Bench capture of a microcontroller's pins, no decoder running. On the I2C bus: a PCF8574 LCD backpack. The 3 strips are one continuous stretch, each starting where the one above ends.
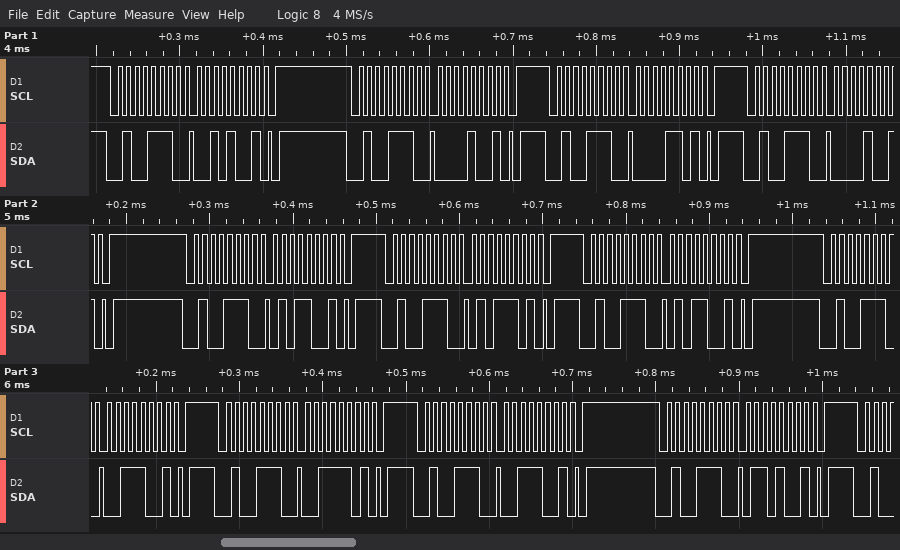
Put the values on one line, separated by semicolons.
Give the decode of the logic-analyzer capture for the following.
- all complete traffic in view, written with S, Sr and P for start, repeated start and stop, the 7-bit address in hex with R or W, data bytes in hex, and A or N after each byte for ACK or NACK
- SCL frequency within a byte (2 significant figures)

S 27W A 29 A P S 27W A 09 A P S 27W A 0D A P S 27W A 09 A P S 27W A 59 A P S 27W A 5D A P S 27W A 59 A P S 27W A 39 A P S 27W A 3D A P S 27W A 39 A P S 27W A 69 A P; 100 kHz
